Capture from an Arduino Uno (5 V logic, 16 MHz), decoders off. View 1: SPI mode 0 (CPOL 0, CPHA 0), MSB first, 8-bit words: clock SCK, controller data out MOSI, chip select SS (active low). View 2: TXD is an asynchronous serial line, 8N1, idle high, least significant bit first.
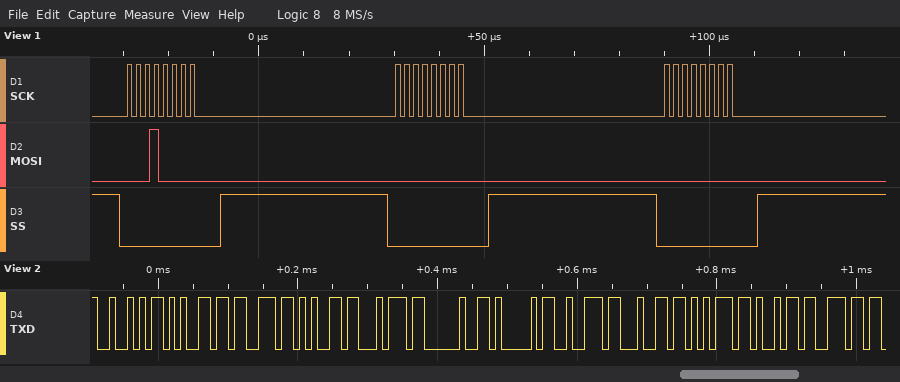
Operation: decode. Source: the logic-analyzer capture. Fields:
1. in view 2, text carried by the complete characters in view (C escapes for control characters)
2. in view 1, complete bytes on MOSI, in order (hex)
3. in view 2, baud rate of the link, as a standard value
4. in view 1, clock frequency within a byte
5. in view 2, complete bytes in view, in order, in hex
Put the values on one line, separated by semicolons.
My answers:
"Reset Arduin"; 0x10 0x00 0x00; 115200 baud; 500 kHz; 52 65 73 65 74 20 41 72 64 75 69 6E
